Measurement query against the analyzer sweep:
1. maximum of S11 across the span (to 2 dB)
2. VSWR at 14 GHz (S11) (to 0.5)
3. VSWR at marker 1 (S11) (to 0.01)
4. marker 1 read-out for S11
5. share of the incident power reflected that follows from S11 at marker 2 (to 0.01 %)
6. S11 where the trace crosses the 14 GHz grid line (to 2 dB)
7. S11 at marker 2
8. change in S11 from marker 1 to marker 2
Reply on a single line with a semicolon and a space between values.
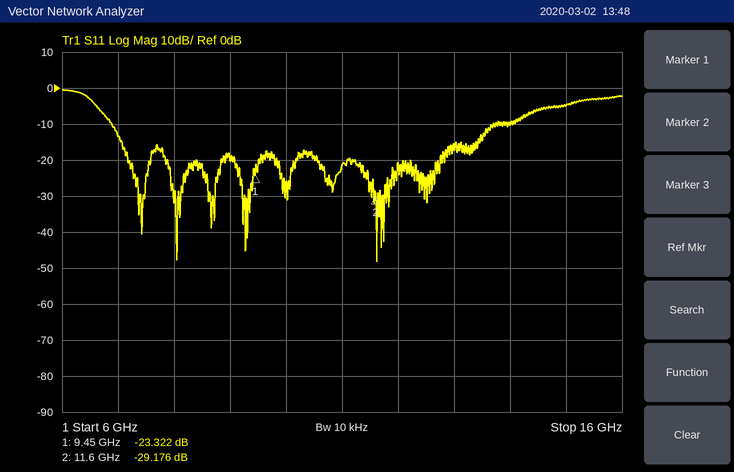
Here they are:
0 dB; 2.0; 1.15; -23.322 dB; 0.12 %; -10 dB; -29.176 dB; -5.854 dB
